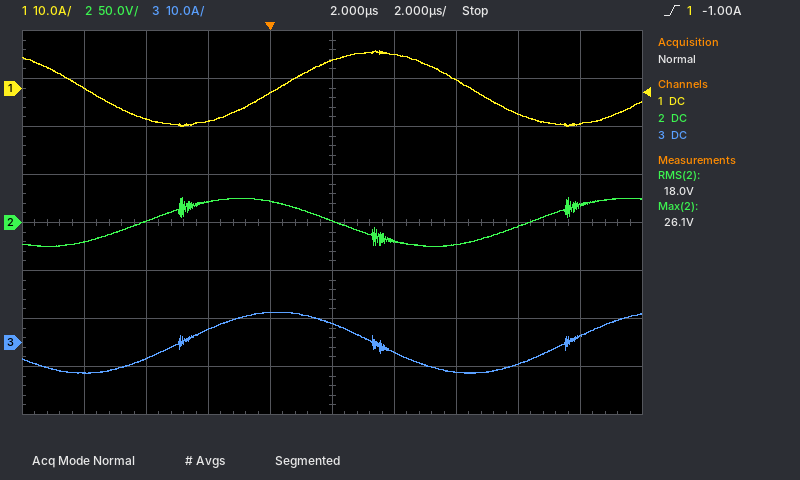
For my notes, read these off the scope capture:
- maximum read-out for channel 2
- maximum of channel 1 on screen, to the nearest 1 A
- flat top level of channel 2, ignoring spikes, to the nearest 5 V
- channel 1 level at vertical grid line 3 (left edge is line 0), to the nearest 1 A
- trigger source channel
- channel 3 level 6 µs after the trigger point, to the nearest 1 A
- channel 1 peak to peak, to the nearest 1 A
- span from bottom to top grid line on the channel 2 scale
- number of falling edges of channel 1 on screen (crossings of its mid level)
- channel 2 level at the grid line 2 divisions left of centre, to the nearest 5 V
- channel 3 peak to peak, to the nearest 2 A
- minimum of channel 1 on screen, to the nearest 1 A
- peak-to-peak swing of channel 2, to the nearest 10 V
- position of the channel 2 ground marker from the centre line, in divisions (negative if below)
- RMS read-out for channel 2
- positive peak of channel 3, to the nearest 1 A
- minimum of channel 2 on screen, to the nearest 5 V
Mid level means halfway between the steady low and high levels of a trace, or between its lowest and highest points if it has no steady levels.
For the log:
26.1 V
8 A
25 V
-7 A
channel 1
-6 A
16 A
400 V
2
20 V
12 A
-8 A
50 V
0.0 div
18.0 V
6 A
-25 V
